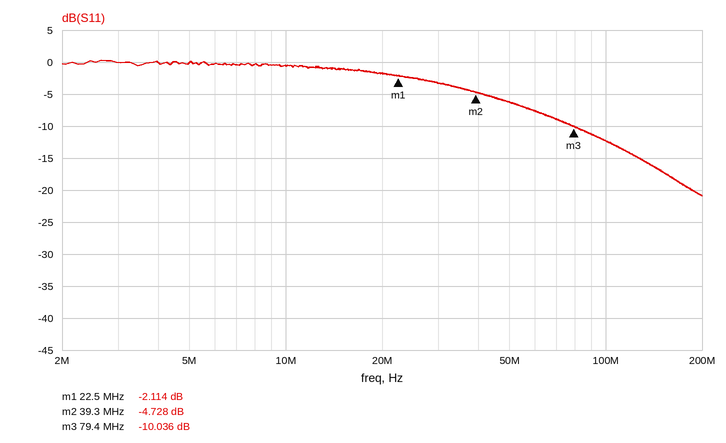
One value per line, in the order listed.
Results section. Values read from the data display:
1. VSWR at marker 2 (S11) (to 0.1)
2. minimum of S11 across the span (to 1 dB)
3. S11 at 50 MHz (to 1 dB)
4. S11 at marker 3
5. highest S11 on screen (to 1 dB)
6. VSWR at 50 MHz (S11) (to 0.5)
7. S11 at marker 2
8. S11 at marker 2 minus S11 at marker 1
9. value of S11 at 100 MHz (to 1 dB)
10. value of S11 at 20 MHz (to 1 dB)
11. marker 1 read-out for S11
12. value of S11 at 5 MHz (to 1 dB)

3.8
-21 dB
-6 dB
-10.036 dB
0 dB
3.0
-4.728 dB
-2.614 dB
-12 dB
-2 dB
-2.114 dB
0 dB
